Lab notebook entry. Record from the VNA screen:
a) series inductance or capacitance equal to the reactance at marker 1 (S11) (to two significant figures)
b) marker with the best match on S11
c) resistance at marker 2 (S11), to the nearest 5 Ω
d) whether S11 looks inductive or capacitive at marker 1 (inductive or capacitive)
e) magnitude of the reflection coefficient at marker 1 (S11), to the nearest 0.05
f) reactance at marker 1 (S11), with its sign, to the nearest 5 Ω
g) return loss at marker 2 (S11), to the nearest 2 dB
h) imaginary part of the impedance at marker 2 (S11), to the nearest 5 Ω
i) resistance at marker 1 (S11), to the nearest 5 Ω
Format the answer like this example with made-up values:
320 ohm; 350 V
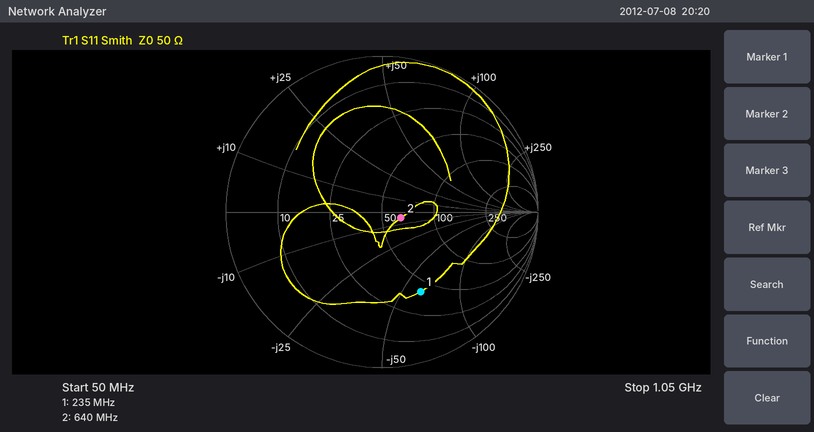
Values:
11 pF; marker 2; 65 Ω; capacitive; 0.55; -60 Ω; 18 dB; -5 Ω; 40 Ω
